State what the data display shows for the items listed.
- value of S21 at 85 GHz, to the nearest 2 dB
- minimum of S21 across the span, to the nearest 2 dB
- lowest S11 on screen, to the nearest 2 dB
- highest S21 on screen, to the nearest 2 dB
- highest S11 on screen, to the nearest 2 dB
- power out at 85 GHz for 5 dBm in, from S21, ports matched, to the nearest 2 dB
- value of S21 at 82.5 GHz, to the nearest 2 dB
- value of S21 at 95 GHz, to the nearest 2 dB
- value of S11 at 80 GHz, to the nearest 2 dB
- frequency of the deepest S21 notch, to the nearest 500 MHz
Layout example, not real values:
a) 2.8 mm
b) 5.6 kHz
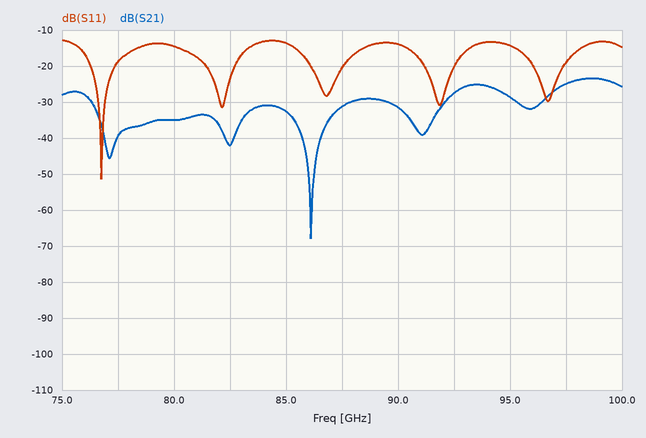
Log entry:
a) -32 dB
b) -68 dB
c) -52 dB
d) -24 dB
e) -12 dB
f) -28 dBm
g) -42 dB
h) -28 dB
i) -14 dB
j) 86.0 GHz
